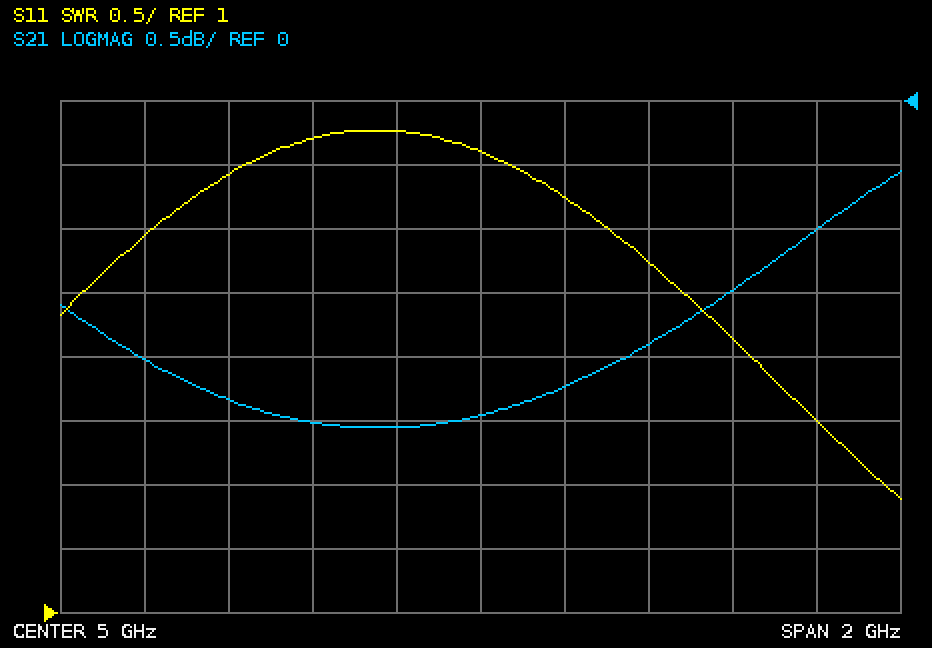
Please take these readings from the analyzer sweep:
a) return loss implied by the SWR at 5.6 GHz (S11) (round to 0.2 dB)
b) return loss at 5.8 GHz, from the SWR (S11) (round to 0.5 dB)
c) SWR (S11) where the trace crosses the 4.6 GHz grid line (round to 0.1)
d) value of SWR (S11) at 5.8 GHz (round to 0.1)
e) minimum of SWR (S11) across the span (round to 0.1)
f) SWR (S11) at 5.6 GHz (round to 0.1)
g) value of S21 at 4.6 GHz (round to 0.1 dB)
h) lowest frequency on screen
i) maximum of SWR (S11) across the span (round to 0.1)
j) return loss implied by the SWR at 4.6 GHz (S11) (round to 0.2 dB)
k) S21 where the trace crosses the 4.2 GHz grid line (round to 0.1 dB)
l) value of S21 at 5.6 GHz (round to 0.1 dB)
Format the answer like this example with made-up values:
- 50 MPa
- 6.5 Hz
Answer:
- 5.8 dB
- 7.5 dB
- 4.7
- 2.5
- 1.9
- 3.1
- -2.5 dB
- 4 GHz
- 4.8
- 3.8 dB
- -2.0 dB
- -1.5 dB
